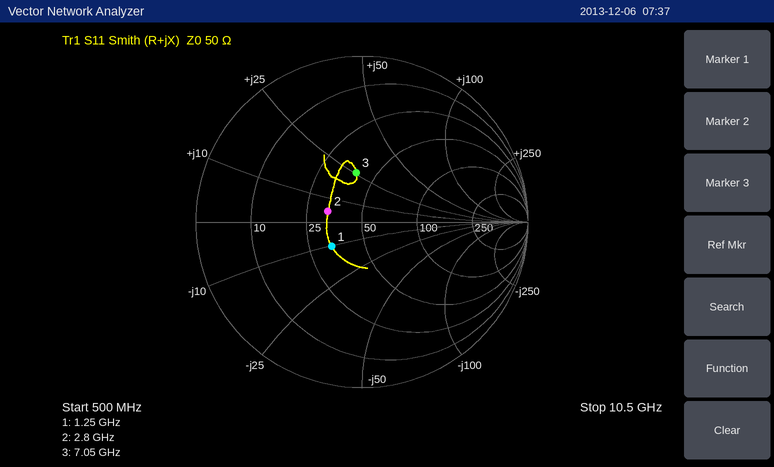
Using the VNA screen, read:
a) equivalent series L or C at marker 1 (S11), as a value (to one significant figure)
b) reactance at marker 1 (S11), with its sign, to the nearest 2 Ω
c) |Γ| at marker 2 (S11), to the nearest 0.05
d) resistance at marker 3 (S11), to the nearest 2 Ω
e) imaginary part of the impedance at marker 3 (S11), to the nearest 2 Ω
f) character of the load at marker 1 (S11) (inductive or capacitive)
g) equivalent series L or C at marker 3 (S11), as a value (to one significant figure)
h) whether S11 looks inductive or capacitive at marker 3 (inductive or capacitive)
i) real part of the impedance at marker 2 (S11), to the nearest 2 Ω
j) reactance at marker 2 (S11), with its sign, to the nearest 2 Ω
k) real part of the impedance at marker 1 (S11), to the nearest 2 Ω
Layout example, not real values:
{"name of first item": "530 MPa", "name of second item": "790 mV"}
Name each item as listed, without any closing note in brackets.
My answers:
{"equivalent series L or C at marker 1 (S11), as a value": "10 pF", "reactance at marker 1 (S11), with its sign, to the nearest 2 Ω": "-10 Ω", "|Γ| at marker 2 (S11), to the nearest 0.05": "0.20", "resistance at marker 3 (S11), to the nearest 2 Ω": "40 Ω", "imaginary part of the impedance at marker 3 (S11), to the nearest 2 Ω": "+26 Ω", "character of the load at marker 1 (S11)": "capacitive", "equivalent series L or C at marker 3 (S11), as a value": "600 pH", "whether S11 looks inductive or capacitive at marker 3": "inductive", "real part of the impedance at marker 2 (S11), to the nearest 2 Ω": "32 Ω", "reactance at marker 2 (S11), with its sign, to the nearest 2 Ω": "+4 Ω", "real part of the impedance at marker 1 (S11), to the nearest 2 Ω": "34 Ω"}
